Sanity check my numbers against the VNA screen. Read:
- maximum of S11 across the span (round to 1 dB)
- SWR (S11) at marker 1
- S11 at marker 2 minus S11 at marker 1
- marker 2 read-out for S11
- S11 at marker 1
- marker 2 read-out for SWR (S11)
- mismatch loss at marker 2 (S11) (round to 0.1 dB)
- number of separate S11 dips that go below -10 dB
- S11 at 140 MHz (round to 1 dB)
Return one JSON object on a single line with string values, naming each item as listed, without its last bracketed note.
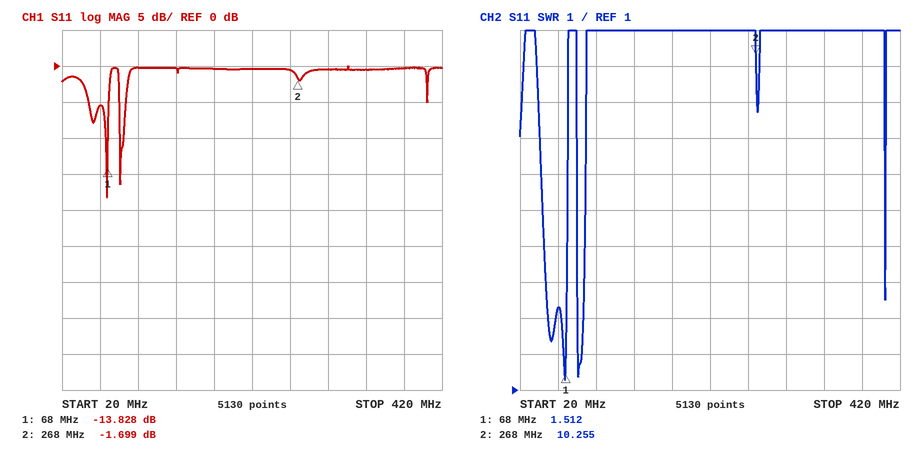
{"maximum of S11 across the span": "0 dB", "SWR (S11) at marker 1": "1.512", "S11 at marker 2 minus S11 at marker 1": "12.129 dB", "marker 2 read-out for S11": "-1.699 dB", "S11 at marker 1": "-13.828 dB", "marker 2 read-out for SWR": "10.255", "mismatch loss at marker 2 (S11)": "4.9 dB", "number of separate S11 dips that go below -10 dB": "2", "S11 at 140 MHz": "0 dB"}
